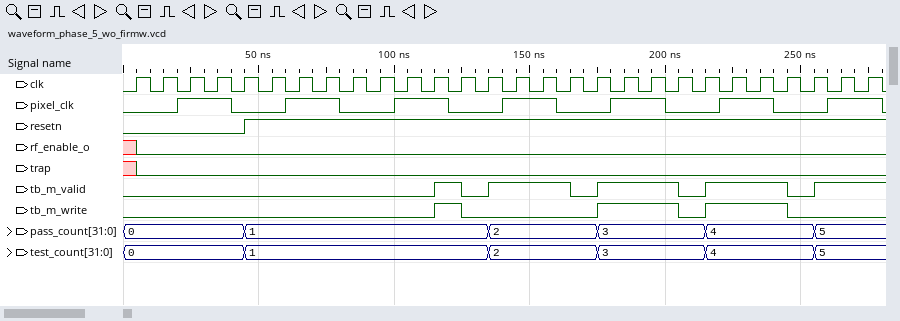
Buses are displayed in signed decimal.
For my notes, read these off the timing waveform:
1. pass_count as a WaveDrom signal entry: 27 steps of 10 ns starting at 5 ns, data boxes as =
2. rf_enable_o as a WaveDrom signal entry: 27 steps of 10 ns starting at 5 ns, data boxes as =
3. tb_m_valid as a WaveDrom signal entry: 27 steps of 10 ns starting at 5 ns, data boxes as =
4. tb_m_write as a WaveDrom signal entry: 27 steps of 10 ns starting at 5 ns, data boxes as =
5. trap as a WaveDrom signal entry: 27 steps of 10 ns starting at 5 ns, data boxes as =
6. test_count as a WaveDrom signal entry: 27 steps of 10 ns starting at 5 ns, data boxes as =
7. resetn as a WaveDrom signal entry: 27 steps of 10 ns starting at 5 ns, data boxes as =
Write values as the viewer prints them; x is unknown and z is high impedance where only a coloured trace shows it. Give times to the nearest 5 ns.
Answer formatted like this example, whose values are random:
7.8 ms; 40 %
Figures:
{name: 'pass_count', wave: '=...=........=...=...=...=.', data: '0 1 2 3 4 5'}; {name: 'rf_enable_o', wave: '0..........................'}; {name: 'tb_m_valid', wave: '0..........101..01..01..01.'}; {name: 'tb_m_write', wave: '0..........10....1..01..0..'}; {name: 'trap', wave: '0..........................'}; {name: 'test_count', wave: '=...=........=...=...=...=.', data: '0 1 2 3 4 5'}; {name: 'resetn', wave: '0...1......................'}
